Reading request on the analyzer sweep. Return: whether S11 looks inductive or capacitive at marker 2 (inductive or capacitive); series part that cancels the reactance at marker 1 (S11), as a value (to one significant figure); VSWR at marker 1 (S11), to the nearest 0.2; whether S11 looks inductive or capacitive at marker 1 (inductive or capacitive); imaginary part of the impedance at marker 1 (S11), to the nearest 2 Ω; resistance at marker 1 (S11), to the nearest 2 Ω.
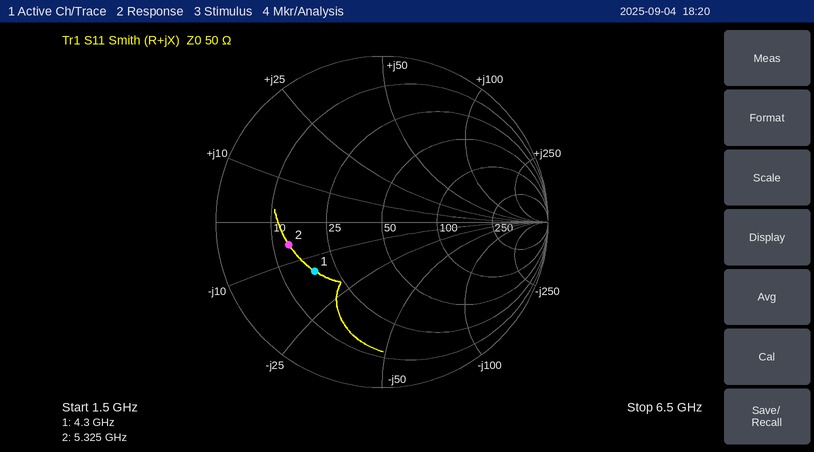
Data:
capacitive
500 pH
3.0
capacitive
-14 Ω
18 Ω
